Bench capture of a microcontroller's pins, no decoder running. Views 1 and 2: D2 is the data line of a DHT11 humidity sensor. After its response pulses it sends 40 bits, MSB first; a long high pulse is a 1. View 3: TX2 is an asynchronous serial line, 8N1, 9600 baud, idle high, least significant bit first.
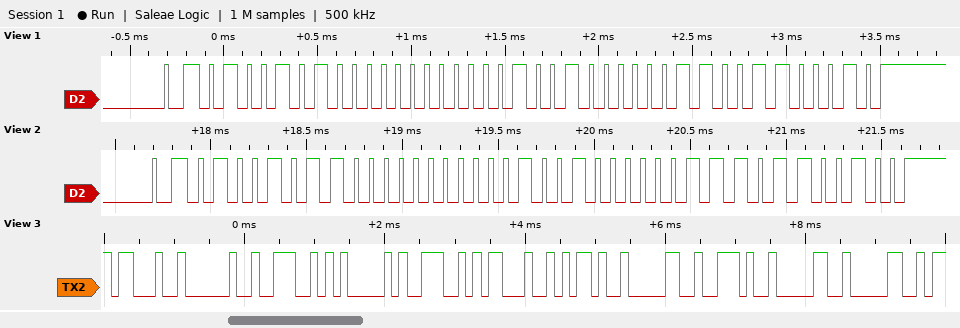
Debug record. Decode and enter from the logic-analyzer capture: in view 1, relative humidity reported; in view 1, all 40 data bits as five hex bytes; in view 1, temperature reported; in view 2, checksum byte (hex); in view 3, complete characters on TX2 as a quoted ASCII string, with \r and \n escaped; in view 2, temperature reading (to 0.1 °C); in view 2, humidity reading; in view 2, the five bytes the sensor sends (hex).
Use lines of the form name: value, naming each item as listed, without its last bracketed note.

in view 1, relative humidity reported: 74 %
in view 1, all 40 data bits as five hex bytes: 4A 00 12 06 62
in view 1, temperature reported: 18.6 °C
in view 2, checksum byte: 0x64
in view 3, complete characters on TX2 as a quoted ASCII string, with \r and \n escaped: "# NAN#-0.00"
in view 2, temperature reading: 18.7 °C
in view 2, humidity reading: 75 %
in view 2, the five bytes the sensor sends: 4B 00 12 07 64
